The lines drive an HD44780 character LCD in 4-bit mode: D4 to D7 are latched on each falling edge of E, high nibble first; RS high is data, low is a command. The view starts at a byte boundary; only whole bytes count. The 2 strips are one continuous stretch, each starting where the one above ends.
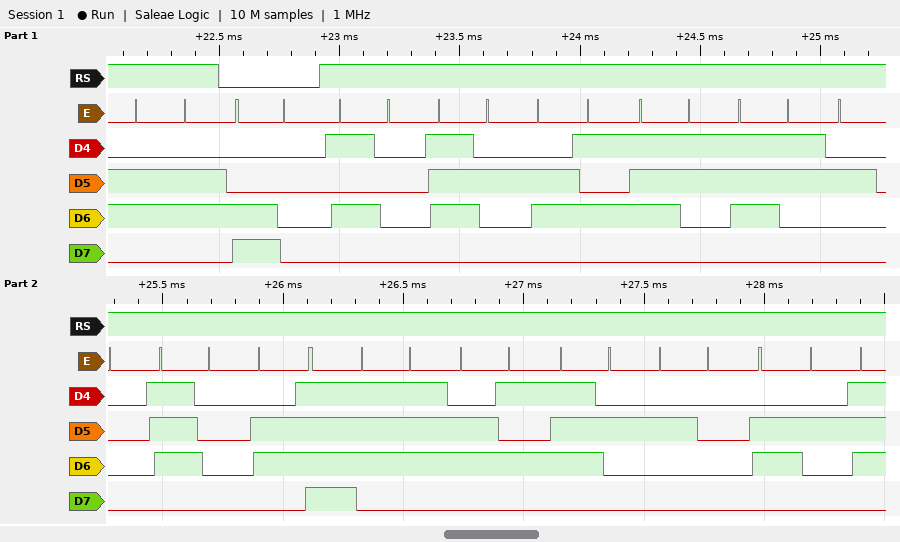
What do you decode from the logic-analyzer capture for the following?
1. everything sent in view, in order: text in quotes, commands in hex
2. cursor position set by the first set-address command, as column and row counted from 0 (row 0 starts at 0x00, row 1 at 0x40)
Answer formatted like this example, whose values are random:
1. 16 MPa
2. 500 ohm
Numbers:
1. "f" 0xC0 "Press power b"
2. column 0, row 1
